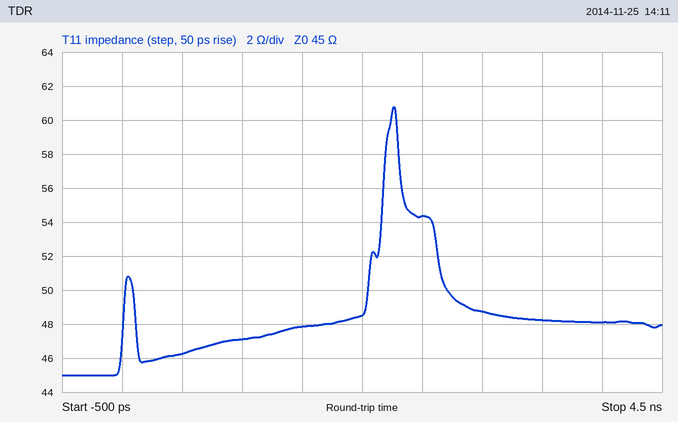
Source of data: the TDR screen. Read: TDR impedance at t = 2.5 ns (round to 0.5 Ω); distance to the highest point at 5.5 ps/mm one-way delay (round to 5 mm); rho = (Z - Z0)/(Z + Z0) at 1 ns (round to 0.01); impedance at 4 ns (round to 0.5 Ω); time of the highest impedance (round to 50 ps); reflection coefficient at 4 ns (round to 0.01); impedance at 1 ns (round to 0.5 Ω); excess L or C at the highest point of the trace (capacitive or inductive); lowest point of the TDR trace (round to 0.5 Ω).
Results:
54.5 Ω
205 mm
+0.02
48.0 Ω
2.25 ns
+0.03
47.0 Ω
inductive
45.0 Ω
